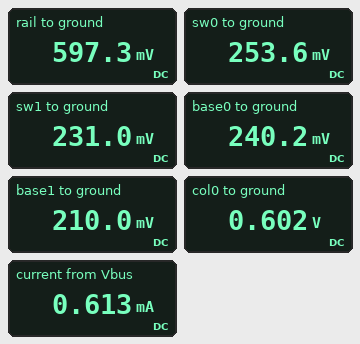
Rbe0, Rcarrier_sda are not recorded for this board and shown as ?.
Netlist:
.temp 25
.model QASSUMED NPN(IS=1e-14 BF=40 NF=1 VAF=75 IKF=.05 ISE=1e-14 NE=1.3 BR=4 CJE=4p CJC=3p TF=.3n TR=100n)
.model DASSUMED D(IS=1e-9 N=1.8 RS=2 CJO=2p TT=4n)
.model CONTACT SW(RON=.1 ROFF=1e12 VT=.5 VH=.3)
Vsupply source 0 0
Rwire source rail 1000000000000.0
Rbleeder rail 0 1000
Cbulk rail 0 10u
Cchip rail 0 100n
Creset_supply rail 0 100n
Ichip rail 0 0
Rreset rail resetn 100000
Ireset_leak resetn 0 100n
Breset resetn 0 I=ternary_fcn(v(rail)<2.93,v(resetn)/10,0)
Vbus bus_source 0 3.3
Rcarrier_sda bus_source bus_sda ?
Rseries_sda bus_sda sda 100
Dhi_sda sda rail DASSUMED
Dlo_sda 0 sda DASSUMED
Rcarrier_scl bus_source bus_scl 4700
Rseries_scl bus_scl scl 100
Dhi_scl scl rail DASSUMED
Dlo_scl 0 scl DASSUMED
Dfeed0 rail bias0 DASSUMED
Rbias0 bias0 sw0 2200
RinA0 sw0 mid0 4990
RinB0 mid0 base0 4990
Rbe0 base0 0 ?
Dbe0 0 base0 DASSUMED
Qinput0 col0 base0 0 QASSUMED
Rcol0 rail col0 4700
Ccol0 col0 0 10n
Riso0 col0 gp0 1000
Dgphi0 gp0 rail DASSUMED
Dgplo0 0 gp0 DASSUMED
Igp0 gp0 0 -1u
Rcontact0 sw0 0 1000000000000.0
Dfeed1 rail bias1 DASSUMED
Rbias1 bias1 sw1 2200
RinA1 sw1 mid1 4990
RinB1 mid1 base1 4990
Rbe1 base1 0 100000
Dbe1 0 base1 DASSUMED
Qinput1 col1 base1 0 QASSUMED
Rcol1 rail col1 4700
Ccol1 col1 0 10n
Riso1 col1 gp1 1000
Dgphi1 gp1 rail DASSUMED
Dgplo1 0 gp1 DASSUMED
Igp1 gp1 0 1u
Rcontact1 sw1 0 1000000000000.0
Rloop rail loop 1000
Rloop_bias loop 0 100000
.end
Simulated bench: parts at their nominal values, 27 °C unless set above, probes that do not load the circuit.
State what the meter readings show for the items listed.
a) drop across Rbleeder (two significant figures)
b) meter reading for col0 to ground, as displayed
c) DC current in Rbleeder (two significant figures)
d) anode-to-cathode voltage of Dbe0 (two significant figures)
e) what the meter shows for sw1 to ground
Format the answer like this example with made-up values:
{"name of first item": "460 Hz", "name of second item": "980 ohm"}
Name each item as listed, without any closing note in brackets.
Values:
{"drop across Rbleeder": "600 mV", "meter reading for col0 to ground, as displayed": "0.602 V", "DC current in Rbleeder": "600 µA", "anode-to-cathode voltage of Dbe0": "-240 mV", "what the meter shows for sw1 to ground": "231.0 mV"}
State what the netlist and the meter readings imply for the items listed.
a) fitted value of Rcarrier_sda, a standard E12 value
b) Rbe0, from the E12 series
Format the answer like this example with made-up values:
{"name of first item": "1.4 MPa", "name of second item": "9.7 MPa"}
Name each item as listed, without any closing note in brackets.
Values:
{"fitted value of Rcarrier_sda, a standard E12 value": "12 kΩ", "Rbe0, from the E12 series": "180 kΩ"}
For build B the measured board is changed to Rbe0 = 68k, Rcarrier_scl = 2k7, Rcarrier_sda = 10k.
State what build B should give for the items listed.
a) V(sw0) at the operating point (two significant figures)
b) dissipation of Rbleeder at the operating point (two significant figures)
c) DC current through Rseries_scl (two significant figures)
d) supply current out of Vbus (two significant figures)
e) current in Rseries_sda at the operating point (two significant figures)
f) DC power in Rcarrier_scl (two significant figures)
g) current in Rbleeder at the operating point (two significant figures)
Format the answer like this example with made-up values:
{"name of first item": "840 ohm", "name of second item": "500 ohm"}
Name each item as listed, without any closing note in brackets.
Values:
{"V(sw0) at the operating point": "410 mV", "dissipation of Rbleeder at the operating point": "680 µW", "DC current through Rseries_scl": "660 µA", "supply current out of Vbus": "850 µA", "current in Rseries_sda at the operating point": "190 µA", "DC power in Rcarrier_scl": "1.2 mW", "current in Rbleeder at the operating point": "820 µA"}
